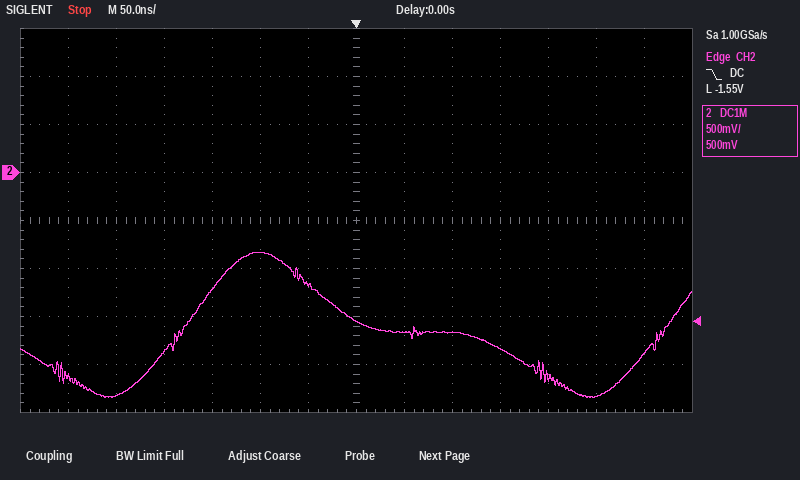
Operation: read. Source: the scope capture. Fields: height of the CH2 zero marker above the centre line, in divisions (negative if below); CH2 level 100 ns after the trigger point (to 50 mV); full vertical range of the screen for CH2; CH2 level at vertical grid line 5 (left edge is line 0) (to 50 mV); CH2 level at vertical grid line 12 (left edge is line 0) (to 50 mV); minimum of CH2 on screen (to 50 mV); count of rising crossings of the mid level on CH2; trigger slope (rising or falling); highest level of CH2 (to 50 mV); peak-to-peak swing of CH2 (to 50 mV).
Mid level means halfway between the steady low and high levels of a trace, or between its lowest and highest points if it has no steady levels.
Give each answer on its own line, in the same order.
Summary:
+1.0 div
-1.65 V
4 V
-850 mV
-2.35 V
-2.35 V
2
falling
-850 mV
1.50 V
